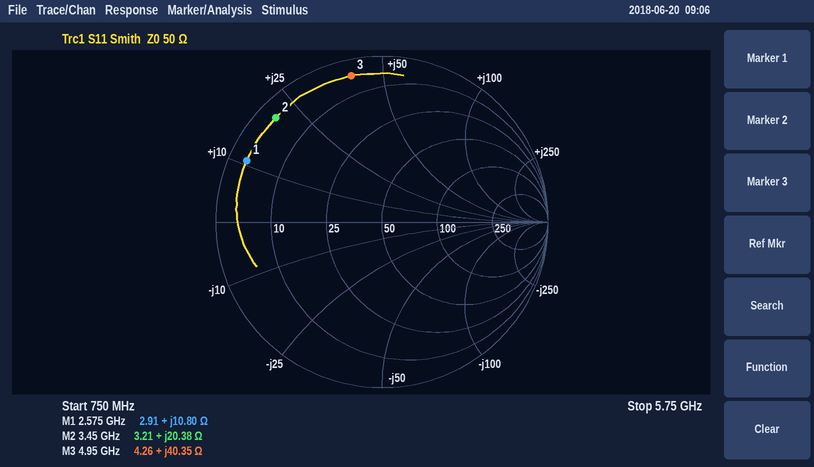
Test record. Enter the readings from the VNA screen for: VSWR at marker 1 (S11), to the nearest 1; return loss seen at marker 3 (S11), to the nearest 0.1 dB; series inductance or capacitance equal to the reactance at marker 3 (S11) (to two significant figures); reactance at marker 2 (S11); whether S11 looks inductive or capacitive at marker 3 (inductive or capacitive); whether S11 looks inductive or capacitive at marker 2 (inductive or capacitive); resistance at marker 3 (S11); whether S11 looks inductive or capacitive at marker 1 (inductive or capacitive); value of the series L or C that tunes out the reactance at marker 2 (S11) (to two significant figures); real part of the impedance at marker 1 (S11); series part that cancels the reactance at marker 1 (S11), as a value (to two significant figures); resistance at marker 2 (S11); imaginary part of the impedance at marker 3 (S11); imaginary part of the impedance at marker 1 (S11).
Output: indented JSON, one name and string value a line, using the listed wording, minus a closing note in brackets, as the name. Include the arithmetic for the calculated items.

{
  "VSWR at marker 1 (S11), to the nearest 1": "18",
  "return loss seen at marker 3 (S11), to the nearest 0.1 dB": "0.9 dB",
  "series inductance or capacitance equal to the reactance at marker 3 (S11)": "L = 40.35 Ω/(2π × 4.95 GHz) ≈ 1.3 nH",
  "reactance at marker 2": "+20.38 Ω",
  "whether S11 looks inductive or capacitive at marker 3": "inductive",
  "whether S11 looks inductive or capacitive at marker 2": "inductive",
  "resistance at marker 3": "4.26 Ω",
  "whether S11 looks inductive or capacitive at marker 1": "inductive",
  "value of the series L or C that tunes out the reactance at marker 2 (S11)": "C = 1/(2π × 3.45 GHz × 20.38 Ω) ≈ 2.3 pF",
  "real part of the impedance at marker 1": "2.91 Ω",
  "series part that cancels the reactance at marker 1 (S11), as a value": "C = 1/(2π × 2.575 GHz × 10.8 Ω) ≈ 5.7 pF",
  "resistance at marker 2": "3.21 Ω",
  "imaginary part of the impedance at marker 3": "+40.35 Ω",
  "imaginary part of the impedance at marker 1": "+10.80 Ω"
}
